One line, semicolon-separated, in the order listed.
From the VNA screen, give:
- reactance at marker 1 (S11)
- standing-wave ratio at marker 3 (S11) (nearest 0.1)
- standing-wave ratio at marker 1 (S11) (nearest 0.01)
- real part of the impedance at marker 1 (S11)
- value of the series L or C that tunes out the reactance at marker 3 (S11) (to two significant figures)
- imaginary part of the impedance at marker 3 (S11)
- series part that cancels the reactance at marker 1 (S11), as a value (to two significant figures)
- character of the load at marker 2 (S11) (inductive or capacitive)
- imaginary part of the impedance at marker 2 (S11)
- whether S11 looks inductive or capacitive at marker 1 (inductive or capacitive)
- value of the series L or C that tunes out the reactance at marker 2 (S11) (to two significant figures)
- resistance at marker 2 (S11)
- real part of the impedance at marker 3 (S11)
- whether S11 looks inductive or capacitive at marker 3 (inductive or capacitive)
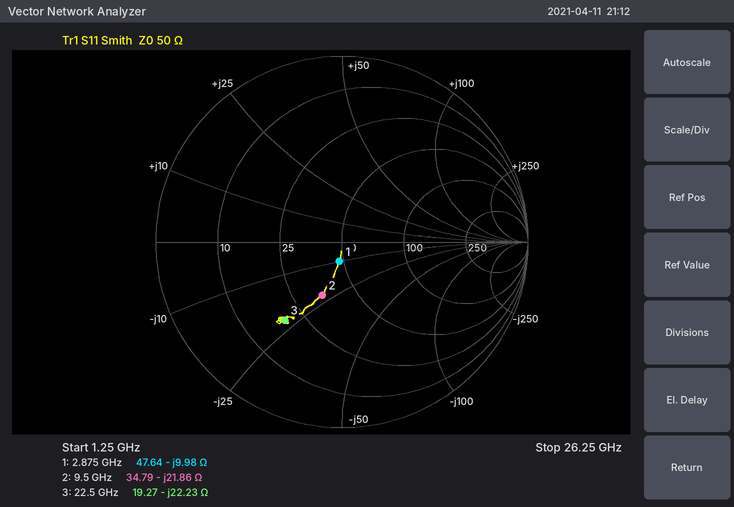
-9.98 Ω; 3.2; 1.23; 47.64 Ω; 160 pH; -22.23 Ω; 550 pH; capacitive; -21.86 Ω; capacitive; 370 pH; 34.79 Ω; 19.27 Ω; capacitive
